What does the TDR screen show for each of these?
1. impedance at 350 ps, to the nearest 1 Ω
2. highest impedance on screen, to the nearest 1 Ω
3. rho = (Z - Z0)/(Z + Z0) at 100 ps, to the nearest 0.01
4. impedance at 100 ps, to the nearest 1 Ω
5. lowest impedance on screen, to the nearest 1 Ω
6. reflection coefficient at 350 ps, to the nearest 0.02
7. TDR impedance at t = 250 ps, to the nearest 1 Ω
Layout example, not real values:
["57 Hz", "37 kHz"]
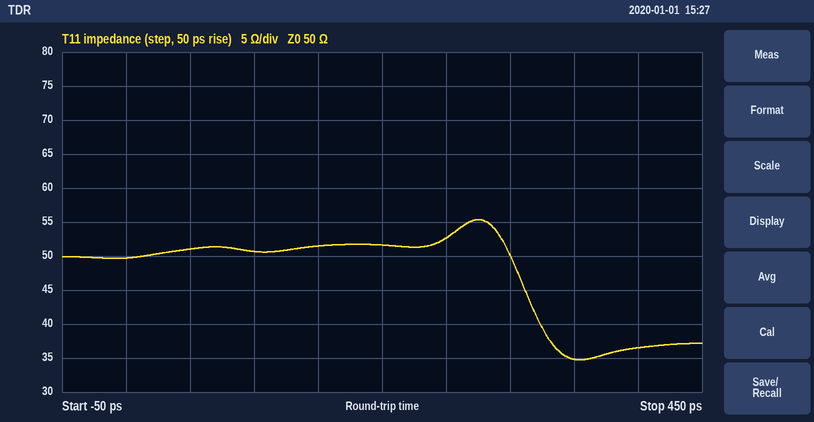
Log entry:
["35 Ω", "55 Ω", "+0.01", "51 Ω", "35 Ω", "-0.18", "53 Ω"]
